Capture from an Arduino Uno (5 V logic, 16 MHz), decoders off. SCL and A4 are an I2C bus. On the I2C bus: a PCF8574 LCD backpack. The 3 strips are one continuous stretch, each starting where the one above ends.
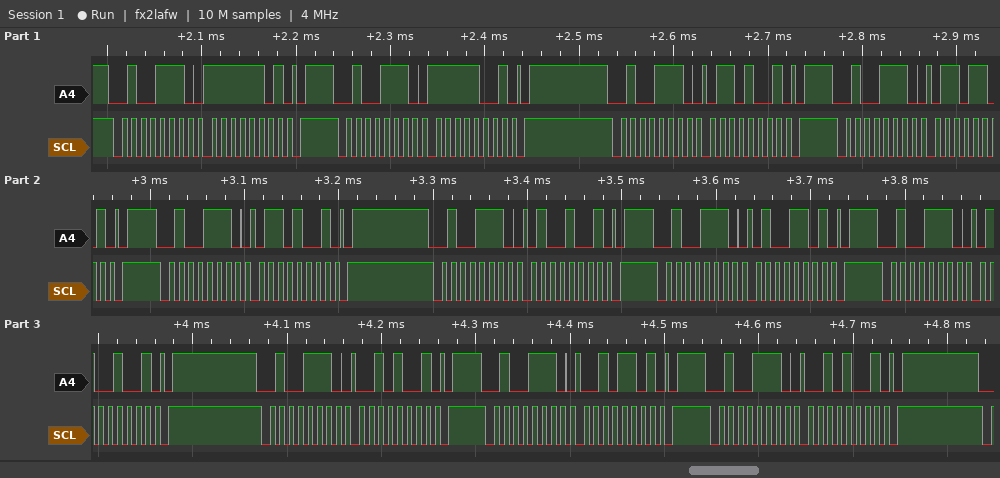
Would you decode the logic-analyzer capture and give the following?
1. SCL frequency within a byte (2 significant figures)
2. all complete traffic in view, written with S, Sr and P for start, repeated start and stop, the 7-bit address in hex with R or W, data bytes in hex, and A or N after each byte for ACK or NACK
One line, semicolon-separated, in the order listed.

100 kHz; S 27W A FD A P S 27W A F9 A P S 27W A 69 A P S 27W A 6D A P S 27W A 69 A P S 27W A 49 A P S 27W A 4D A P S 27W A 49 A P S 27W A 29 A P S 27W A 2D A P S 27W A 29 A P
